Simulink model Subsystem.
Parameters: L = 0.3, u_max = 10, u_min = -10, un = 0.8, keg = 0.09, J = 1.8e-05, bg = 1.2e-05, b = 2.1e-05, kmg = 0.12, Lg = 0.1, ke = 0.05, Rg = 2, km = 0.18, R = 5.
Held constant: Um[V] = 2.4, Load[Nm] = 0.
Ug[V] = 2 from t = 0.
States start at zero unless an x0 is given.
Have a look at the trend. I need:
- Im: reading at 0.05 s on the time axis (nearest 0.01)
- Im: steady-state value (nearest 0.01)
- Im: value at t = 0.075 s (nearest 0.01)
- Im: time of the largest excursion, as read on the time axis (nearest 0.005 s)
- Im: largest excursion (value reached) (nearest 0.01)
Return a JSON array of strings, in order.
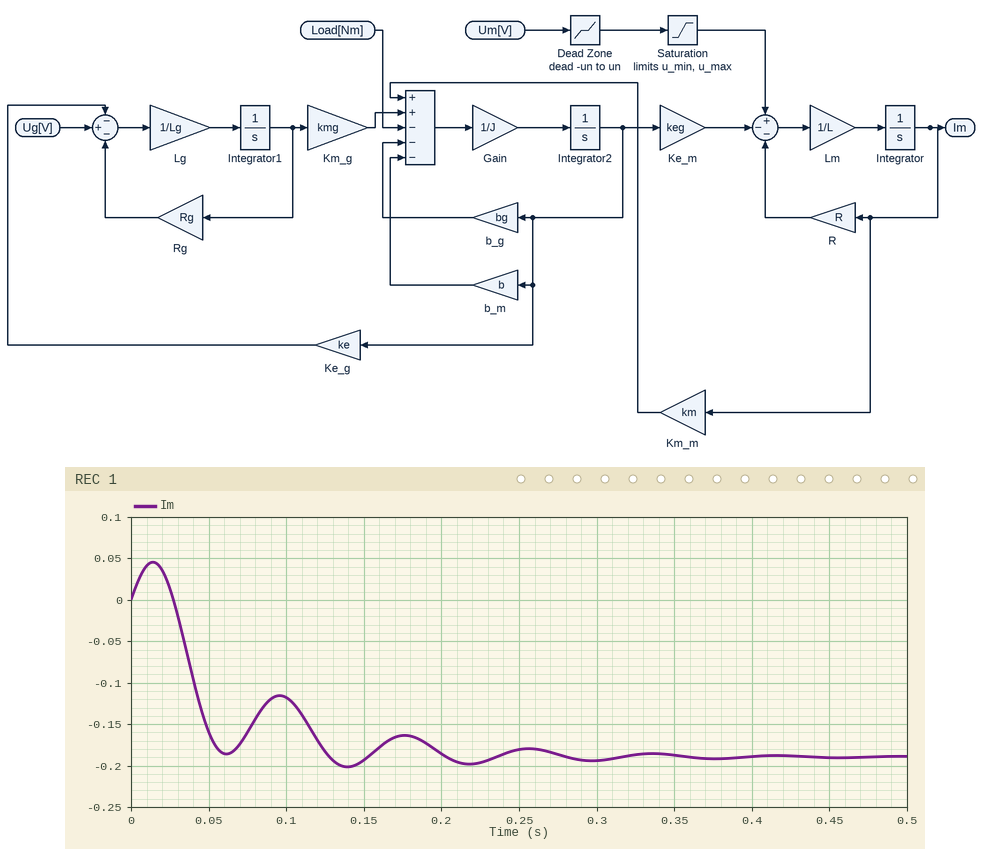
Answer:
["-0.16", "-0.19", "-0.16", "0.140 s", "-0.20"]
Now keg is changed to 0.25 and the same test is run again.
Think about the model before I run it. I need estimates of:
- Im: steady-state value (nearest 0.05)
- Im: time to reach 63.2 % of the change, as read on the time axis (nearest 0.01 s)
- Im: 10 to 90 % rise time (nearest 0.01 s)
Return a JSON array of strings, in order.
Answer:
["-0.40", "0.04 s", "0.07 s"]
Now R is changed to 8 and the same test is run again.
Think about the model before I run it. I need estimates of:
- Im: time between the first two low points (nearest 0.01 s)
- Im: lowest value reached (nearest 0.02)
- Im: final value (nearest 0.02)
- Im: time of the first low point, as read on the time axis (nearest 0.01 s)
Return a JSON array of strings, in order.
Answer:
["0.08 s", "-0.16", "-0.14", "0.06 s"]
